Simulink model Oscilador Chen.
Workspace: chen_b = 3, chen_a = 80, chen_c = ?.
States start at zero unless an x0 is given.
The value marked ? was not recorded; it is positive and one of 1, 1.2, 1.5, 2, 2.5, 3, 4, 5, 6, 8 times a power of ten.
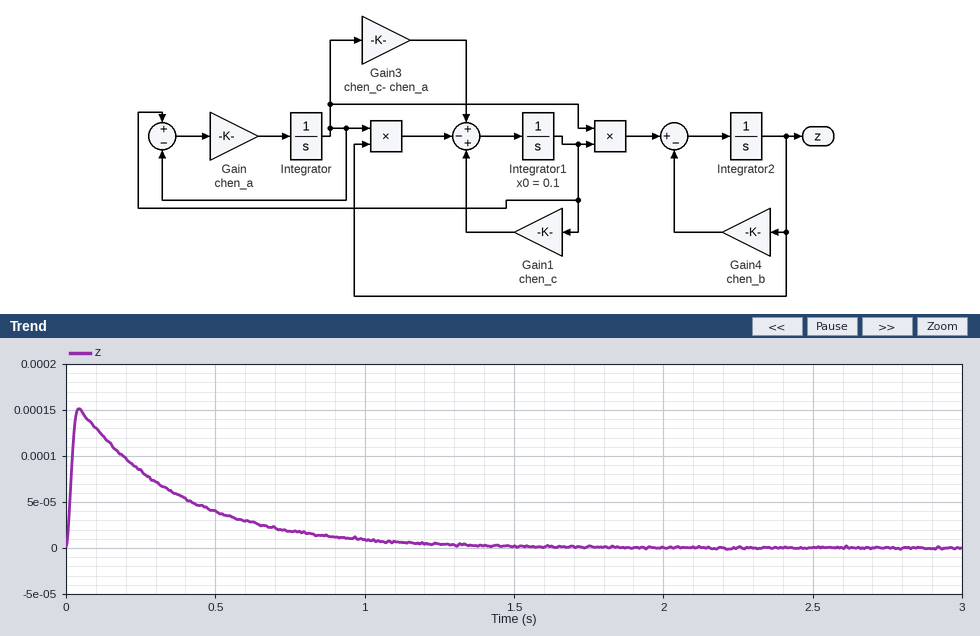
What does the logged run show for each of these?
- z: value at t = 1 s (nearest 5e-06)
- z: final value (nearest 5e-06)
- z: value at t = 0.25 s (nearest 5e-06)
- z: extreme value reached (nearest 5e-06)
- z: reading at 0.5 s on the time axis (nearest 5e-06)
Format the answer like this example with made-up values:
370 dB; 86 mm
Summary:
0.000010; 0.000000; 0.000085; 0.000150; 0.000040
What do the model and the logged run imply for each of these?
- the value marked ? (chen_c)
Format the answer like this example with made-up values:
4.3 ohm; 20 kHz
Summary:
20
